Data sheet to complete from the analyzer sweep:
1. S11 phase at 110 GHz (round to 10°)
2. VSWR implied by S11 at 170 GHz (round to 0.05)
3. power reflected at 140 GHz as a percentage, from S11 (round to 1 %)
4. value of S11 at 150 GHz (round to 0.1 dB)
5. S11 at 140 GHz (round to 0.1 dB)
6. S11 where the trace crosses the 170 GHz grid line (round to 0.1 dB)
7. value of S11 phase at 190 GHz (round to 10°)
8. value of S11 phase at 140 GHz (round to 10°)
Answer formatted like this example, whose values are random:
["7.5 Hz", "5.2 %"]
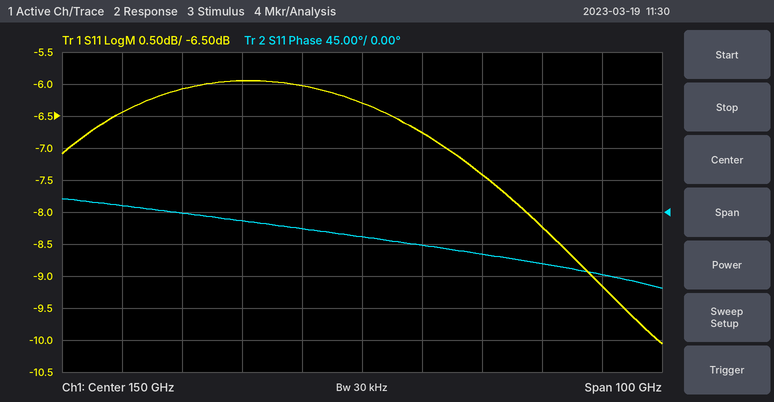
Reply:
["10°", "2.50", "25 %", "-6.3 dB", "-6.0 dB", "-7.4 dB", "-90°", "-20°"]
